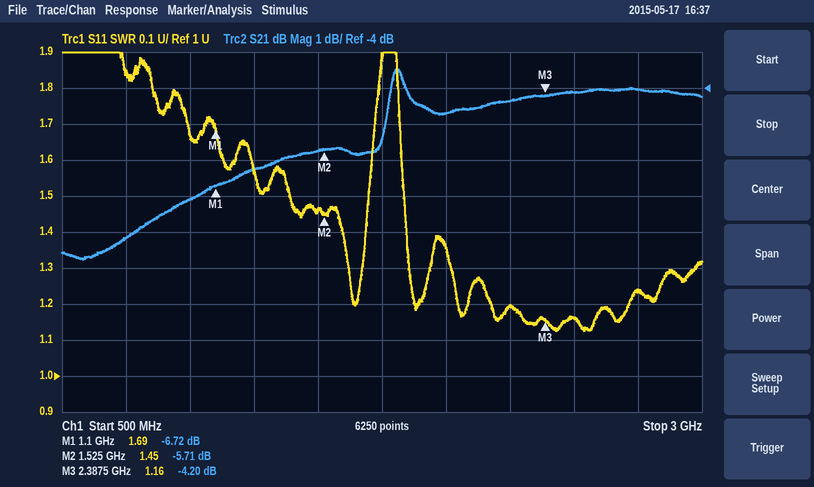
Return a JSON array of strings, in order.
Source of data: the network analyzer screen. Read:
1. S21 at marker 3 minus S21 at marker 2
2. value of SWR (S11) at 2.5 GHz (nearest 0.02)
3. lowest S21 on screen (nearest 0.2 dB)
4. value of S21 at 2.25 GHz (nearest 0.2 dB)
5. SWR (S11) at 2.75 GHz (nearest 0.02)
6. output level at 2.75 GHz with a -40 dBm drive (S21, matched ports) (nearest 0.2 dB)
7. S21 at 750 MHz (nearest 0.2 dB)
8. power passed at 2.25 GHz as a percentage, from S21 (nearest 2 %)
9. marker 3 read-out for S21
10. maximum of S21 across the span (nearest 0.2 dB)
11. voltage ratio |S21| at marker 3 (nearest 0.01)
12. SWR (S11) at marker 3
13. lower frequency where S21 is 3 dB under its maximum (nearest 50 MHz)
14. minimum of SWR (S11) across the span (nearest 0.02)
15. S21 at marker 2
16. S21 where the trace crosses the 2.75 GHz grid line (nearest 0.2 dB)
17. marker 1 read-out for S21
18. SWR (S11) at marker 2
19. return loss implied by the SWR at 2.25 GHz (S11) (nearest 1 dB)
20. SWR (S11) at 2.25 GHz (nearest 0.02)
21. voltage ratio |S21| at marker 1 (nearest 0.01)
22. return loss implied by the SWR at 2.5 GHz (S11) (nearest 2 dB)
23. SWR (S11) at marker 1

["1.51 dB", "1.16", "-8.8 dB", "-4.4 dB", "1.24", "-44.0 dBm", "-8.2 dB", "36 %", "-4.20 dB", "-3.4 dB", "0.62", "1.16", "1.20 GHz", "1.12", "-5.71 dB", "-4.0 dB", "-6.72 dB", "1.45", "21 dB", "1.20", "0.46", "22 dB", "1.69"]
